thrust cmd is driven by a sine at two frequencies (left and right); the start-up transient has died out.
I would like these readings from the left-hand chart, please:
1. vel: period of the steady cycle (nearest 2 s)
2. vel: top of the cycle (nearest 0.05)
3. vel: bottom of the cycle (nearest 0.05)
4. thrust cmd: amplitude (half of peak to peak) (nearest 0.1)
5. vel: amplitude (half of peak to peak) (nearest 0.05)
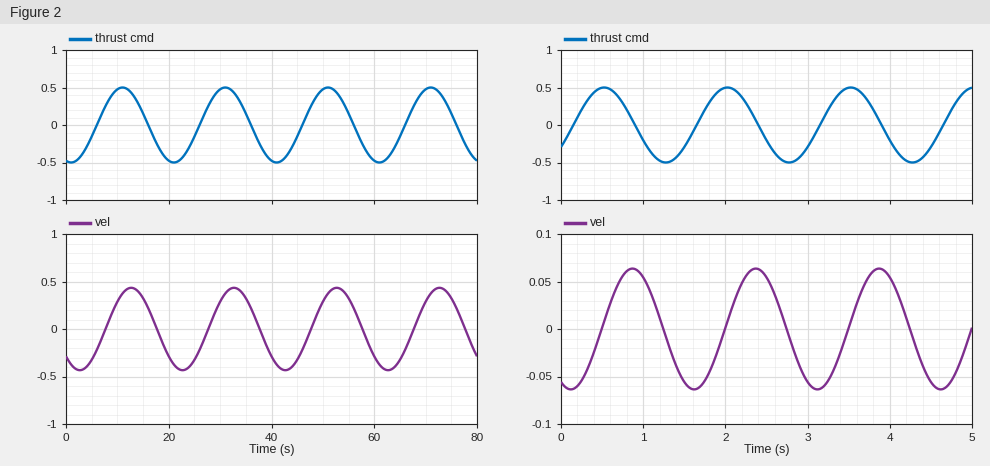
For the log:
20 s
0.45
-0.45
0.5
0.45
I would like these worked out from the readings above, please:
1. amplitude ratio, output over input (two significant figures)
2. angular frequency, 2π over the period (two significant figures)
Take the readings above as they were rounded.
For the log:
0.90
0.31 rad/s
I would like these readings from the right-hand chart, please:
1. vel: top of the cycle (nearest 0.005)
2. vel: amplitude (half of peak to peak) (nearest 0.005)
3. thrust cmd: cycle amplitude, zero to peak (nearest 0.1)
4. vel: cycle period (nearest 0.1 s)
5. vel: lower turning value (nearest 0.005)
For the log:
0.065
0.065
0.5
1.5 s
-0.065
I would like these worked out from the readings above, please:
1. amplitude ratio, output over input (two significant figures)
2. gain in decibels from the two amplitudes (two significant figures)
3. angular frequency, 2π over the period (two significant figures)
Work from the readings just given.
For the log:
0.13
-18 dB
4.2 rad/s
